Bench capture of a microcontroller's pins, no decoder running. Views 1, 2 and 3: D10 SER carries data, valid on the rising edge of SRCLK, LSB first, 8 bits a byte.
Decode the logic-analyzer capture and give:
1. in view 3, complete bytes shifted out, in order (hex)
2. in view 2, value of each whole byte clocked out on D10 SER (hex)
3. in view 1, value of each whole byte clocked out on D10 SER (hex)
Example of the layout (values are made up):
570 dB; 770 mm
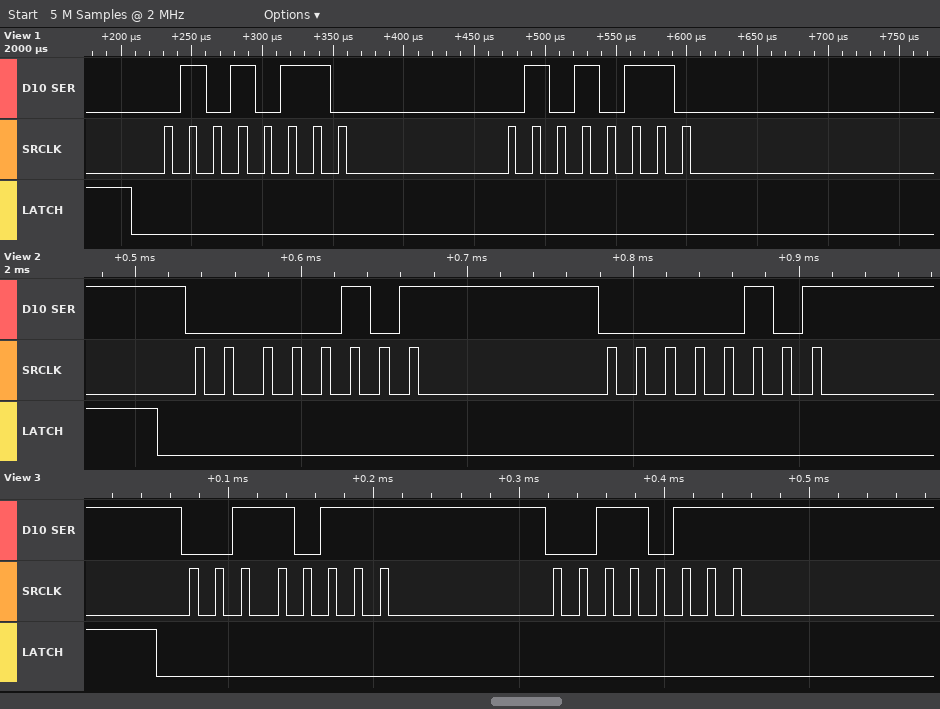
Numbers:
EC EC; A0 A0; 6A 6A
